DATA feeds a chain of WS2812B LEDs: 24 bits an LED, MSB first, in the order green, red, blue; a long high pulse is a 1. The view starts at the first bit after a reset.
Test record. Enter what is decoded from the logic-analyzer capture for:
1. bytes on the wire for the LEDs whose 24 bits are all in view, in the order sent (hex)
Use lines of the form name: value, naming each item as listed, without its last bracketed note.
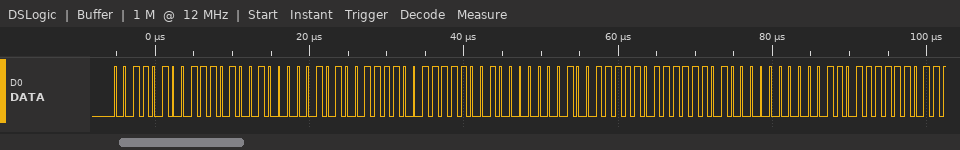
bytes on the wire for the LEDs whose 24 bits are all in view, in the order sent: 34 E9 05 3C F9 01 3E FD 00
